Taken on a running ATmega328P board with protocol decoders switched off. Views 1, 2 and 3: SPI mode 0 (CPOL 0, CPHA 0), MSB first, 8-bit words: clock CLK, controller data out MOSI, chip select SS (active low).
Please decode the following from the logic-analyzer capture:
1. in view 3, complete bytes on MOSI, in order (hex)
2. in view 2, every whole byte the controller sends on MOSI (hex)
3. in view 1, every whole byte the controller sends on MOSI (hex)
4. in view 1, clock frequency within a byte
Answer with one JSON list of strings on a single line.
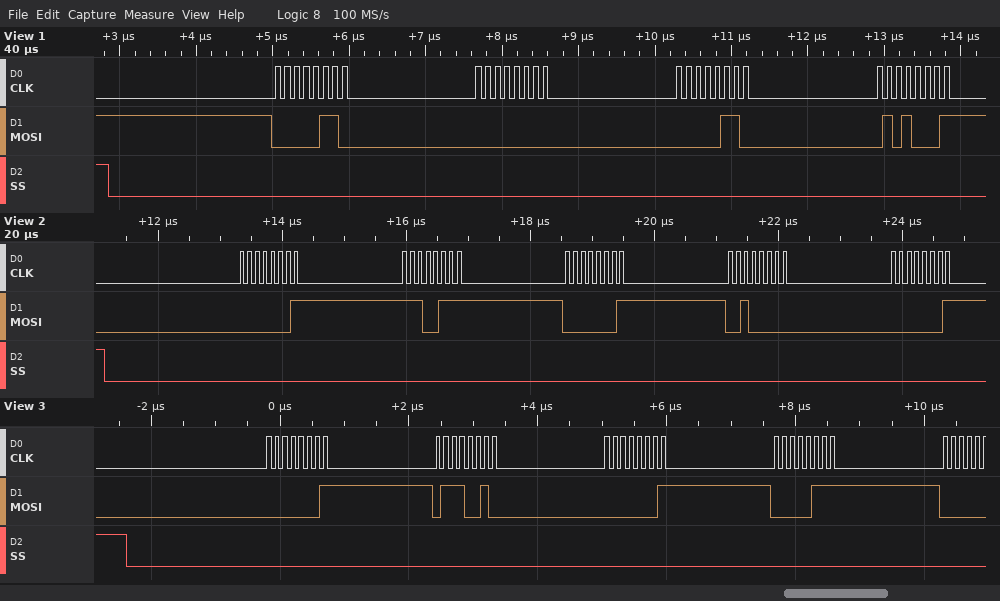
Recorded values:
["01 72 01 07", "01 E7 01 20 01", "0x06 0x00 0x06 0x51", "8 MHz"]
